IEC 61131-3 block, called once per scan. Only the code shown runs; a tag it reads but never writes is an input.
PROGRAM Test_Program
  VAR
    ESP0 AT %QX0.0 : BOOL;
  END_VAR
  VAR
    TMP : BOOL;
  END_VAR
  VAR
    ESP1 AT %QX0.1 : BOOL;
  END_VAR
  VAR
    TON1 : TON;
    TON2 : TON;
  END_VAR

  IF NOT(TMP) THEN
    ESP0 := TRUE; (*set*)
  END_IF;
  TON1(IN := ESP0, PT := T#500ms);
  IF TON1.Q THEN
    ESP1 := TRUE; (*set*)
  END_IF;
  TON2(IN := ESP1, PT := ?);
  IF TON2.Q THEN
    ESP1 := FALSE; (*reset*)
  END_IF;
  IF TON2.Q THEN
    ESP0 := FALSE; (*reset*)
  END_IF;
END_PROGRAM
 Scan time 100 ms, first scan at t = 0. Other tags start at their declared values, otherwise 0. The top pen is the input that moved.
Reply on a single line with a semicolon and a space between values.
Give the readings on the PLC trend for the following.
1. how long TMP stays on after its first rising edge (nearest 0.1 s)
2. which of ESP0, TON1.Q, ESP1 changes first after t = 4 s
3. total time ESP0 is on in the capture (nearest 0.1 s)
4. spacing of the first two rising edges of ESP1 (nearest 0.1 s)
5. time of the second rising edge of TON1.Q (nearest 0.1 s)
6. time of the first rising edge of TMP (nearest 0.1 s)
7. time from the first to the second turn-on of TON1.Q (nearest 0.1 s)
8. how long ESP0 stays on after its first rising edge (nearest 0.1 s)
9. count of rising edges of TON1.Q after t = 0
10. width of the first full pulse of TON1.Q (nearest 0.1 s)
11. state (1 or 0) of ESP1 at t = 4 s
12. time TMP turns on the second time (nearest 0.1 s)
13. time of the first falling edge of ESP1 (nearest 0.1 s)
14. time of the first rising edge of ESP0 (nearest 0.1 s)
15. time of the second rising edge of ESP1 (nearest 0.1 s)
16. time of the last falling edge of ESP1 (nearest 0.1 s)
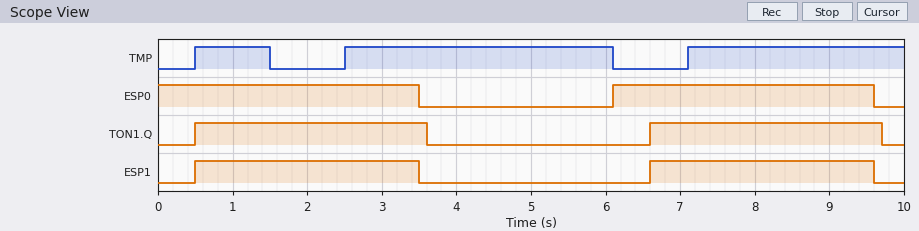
1.0 s; ESP0; 7.0 s; 6.1 s; 6.6 s; 0.5 s; 6.1 s; 3.5 s; 2; 3.1 s; 0; 2.5 s; 3.5 s; 6.1 s; 6.6 s; 9.6 s
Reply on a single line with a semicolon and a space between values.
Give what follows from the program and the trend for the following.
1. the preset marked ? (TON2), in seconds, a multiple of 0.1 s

3.0 s
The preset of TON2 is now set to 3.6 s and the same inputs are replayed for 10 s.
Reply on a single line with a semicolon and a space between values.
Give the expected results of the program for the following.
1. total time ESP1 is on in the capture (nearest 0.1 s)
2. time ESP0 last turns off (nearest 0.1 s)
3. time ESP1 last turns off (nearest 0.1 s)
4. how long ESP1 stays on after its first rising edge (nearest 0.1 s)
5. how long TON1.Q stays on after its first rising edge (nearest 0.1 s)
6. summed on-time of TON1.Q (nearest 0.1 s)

7.0 s; 4.1 s; 4.1 s; 3.6 s; 3.7 s; 7.1 s
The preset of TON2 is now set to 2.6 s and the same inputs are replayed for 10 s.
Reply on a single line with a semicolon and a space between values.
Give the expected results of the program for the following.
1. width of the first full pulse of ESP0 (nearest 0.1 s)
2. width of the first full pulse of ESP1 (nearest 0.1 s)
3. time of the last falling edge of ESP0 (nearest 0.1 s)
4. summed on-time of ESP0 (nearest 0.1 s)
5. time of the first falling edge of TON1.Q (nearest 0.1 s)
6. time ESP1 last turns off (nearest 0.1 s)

3.1 s; 2.6 s; 9.2 s; 6.2 s; 3.2 s; 9.2 s
